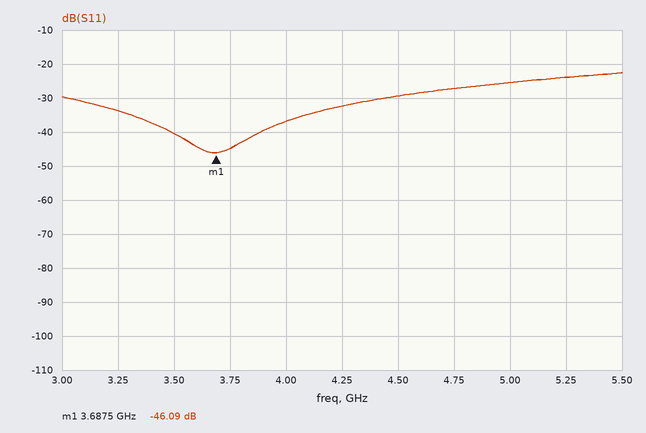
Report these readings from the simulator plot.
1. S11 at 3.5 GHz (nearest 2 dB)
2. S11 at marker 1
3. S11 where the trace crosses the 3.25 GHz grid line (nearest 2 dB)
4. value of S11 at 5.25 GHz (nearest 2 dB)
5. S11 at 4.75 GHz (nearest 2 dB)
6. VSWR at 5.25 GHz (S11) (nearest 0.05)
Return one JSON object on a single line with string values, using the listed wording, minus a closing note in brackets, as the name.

{"S11 at 3.5 GHz": "-40 dB", "S11 at marker 1": "-46.09 dB", "S11 where the trace crosses the 3.25 GHz grid line": "-34 dB", "value of S11 at 5.25 GHz": "-24 dB", "S11 at 4.75 GHz": "-28 dB", "VSWR at 5.25 GHz (S11)": "1.15"}
